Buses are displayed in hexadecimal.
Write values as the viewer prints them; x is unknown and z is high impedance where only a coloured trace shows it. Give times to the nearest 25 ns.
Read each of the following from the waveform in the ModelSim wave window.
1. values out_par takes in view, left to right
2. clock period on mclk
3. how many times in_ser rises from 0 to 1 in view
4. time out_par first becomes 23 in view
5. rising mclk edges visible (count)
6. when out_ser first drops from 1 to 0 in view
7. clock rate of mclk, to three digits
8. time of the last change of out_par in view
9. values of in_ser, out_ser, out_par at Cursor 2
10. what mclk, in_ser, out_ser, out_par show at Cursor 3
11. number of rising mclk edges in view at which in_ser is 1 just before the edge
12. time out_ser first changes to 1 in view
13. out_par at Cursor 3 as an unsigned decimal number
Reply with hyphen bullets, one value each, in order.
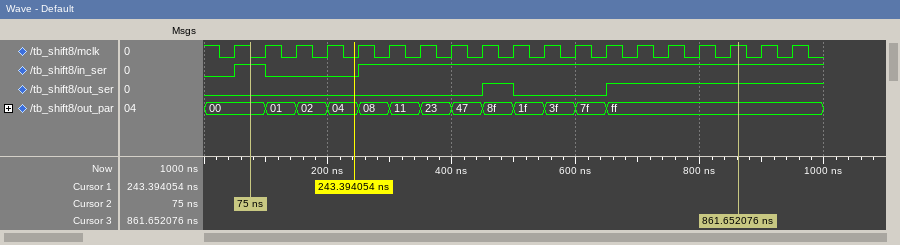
- 00, 01, 02, 04, 08, 11, 23, 47, 8f, 1f, 3f, 7f, ff
- 50 ns
- 2
- 350 ns
- 19
- 500 ns
- 20.0 MHz
- 650 ns
- in_ser=1, out_ser=0, out_par=00
- mclk=1, in_ser=1, out_ser=1, out_par=ff
- 15
- 450 ns
- 255
